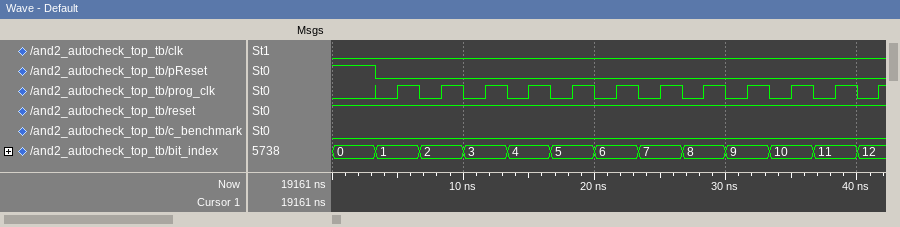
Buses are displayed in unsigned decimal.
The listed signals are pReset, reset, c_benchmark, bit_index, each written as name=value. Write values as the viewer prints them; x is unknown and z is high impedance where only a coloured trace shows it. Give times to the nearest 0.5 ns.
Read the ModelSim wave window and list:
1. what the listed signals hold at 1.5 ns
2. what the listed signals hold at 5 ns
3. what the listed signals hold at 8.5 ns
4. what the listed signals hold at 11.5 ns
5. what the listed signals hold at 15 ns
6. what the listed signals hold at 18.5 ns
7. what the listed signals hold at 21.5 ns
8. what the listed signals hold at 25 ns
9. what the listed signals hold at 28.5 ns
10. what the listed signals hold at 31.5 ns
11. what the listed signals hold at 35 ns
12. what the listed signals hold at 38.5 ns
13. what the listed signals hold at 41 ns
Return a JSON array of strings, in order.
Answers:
["pReset=1, reset=1, c_benchmark=0, bit_index=0", "pReset=0, reset=1, c_benchmark=0, bit_index=1", "pReset=0, reset=1, c_benchmark=0, bit_index=2", "pReset=0, reset=1, c_benchmark=0, bit_index=3", "pReset=0, reset=1, c_benchmark=0, bit_index=4", "pReset=0, reset=1, c_benchmark=0, bit_index=5", "pReset=0, reset=1, c_benchmark=0, bit_index=6", "pReset=0, reset=1, c_benchmark=0, bit_index=7", "pReset=0, reset=1, c_benchmark=0, bit_index=8", "pReset=0, reset=1, c_benchmark=0, bit_index=9", "pReset=0, reset=1, c_benchmark=0, bit_index=10", "pReset=0, reset=1, c_benchmark=0, bit_index=11", "pReset=0, reset=1, c_benchmark=0, bit_index=12"]
